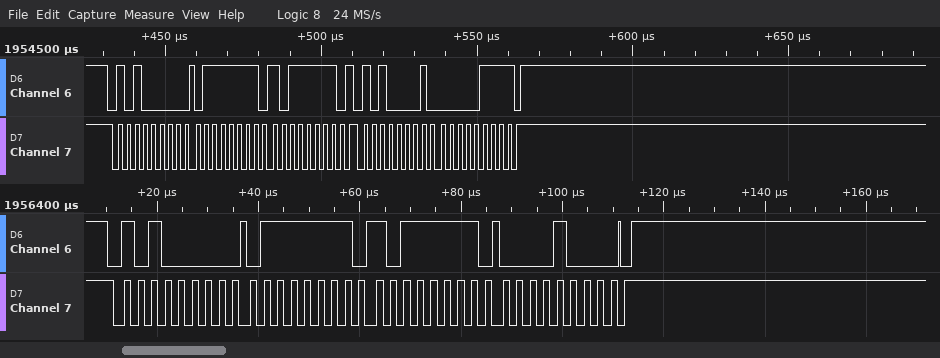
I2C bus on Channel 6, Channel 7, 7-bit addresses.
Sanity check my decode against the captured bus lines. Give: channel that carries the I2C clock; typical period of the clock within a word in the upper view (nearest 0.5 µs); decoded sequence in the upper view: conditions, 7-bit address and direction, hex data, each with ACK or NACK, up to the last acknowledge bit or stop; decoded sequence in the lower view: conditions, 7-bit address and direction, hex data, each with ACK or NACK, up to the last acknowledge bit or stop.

Channel 7
2.5 µs
start, address 50 write ACK, 7F ACK, BF ACK, repeated start, address 50 read ACK, 07 NACK, stop
start, address 50 write ACK, 7F ACK, BF ACK, 08 ACK, stop
